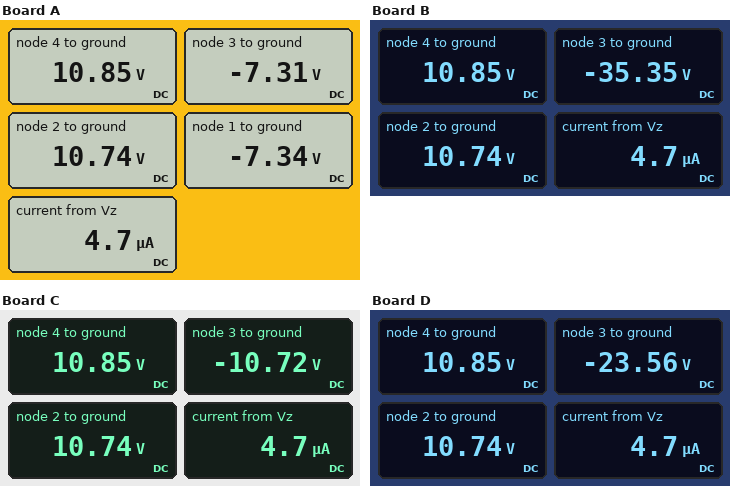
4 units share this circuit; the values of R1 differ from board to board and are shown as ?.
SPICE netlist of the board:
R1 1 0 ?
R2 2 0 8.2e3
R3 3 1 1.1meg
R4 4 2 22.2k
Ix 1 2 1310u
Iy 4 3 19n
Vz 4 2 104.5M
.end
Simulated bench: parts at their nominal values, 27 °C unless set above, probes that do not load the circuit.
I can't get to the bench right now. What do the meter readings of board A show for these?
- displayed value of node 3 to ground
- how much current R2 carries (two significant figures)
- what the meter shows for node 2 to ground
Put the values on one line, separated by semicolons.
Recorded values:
-7.31 V; 1.3 mA; 10.74 V
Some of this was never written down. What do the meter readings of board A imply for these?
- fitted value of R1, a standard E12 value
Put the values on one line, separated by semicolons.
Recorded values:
5.6 kΩ
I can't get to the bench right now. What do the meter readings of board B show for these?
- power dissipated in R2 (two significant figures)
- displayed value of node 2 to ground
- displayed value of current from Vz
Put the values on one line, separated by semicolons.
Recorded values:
14 mW; 10.74 V; 4.7 µA
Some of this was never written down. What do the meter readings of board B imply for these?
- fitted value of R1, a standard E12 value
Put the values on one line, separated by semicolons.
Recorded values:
27 kΩ
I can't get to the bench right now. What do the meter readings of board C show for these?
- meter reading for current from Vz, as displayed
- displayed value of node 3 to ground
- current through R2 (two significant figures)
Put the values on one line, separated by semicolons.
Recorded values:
4.7 µA; -10.72 V; 1.3 mA
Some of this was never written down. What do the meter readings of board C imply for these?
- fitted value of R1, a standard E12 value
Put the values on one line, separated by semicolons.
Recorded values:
8.2 kΩ
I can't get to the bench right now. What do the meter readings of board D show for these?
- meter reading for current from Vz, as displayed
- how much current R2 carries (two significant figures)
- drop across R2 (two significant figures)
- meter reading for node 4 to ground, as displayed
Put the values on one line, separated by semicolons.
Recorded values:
4.7 µA; 1.3 mA; 11 V; 10.85 V
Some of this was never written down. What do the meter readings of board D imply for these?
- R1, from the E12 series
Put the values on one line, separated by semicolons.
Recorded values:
18 kΩ
